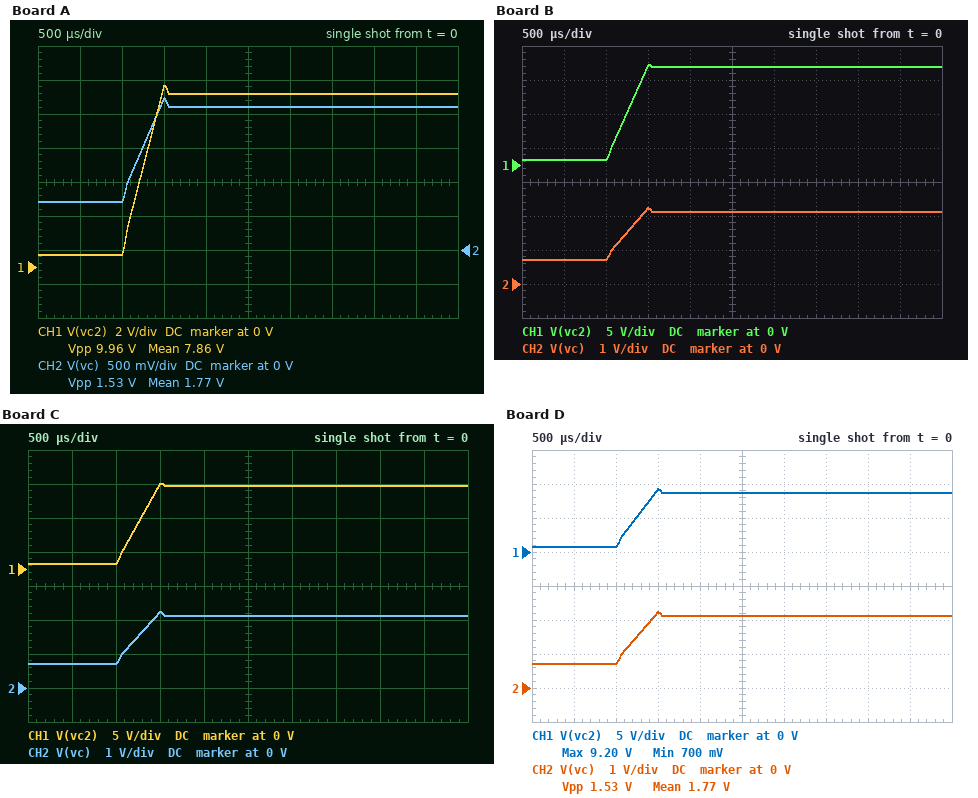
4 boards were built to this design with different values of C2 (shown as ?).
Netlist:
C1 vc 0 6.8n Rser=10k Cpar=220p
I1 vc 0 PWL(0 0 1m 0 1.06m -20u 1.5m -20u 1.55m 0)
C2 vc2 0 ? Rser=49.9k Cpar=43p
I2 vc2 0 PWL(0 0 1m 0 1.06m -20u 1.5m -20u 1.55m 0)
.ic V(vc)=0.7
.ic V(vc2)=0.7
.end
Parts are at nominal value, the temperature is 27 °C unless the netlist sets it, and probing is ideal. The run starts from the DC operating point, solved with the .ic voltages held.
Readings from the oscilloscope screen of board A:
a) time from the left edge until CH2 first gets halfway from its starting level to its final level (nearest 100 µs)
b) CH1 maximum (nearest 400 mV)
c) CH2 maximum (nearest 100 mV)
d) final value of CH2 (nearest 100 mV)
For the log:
1.2 ms
10.8 V
2.2 V
2.1 V
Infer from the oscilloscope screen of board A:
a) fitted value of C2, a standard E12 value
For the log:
1 nF
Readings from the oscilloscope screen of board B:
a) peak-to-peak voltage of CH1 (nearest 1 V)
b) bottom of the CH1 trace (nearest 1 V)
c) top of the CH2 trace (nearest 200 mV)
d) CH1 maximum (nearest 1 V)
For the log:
14 V
1 V
2.2 V
15 V
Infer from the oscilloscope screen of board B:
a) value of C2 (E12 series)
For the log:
680 pF
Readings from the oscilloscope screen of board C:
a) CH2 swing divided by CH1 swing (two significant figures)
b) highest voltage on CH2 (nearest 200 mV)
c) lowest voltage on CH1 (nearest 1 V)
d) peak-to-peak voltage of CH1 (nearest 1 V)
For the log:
0.13
2.2 V
1 V
12 V
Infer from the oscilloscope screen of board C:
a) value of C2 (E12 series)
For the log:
820 pF
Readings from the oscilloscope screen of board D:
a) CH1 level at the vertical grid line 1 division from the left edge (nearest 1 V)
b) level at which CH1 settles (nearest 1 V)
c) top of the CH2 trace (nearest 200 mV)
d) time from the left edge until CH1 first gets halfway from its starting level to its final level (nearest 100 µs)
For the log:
1 V
9 V
2.2 V
1.2 ms
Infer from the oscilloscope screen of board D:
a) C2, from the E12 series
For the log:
1.2 nF
